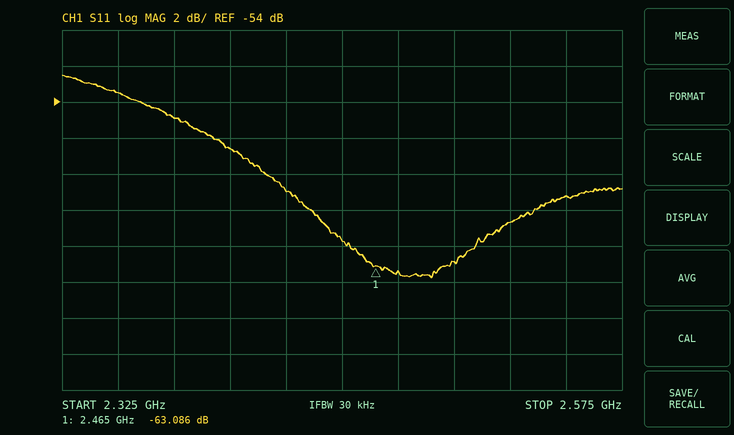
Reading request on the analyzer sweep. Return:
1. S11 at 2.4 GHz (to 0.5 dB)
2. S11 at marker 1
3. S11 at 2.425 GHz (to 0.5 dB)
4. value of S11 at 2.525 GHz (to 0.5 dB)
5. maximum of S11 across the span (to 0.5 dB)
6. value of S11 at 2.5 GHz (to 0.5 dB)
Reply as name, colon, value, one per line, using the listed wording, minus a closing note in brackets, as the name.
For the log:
S11 at 2.4 GHz: -56.5 dB
S11 at marker 1: -63.086 dB
S11 at 2.425 GHz: -59.0 dB
value of S11 at 2.525 GHz: -60.5 dB
maximum of S11 across the span: -52.5 dB
value of S11 at 2.5 GHz: -63.0 dB
